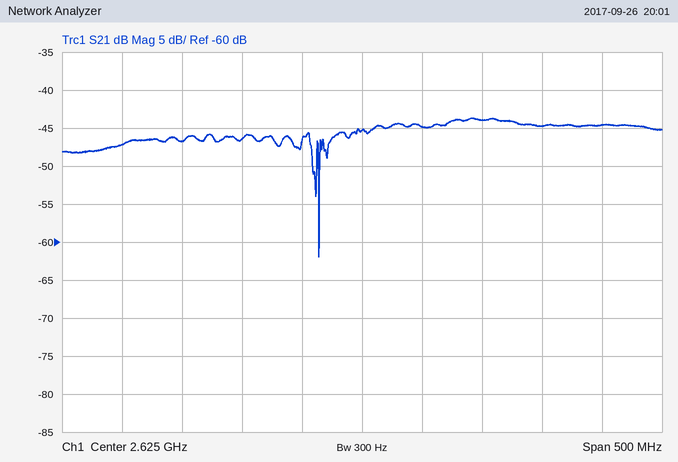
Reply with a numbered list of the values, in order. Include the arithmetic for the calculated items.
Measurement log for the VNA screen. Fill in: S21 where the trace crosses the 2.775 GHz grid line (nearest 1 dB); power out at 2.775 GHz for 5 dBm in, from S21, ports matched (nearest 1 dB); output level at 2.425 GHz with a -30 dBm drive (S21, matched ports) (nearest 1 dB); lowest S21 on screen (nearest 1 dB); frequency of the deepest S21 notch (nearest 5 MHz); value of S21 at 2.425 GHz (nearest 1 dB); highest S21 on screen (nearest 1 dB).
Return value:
1. -45 dB
2. 5 dBm + (-45 dB) = -40 dBm
3. -30 dBm + (-47 dB) = -77 dBm
4. -62 dB
5. 2.590 GHz
6. -47 dB
7. -44 dB
